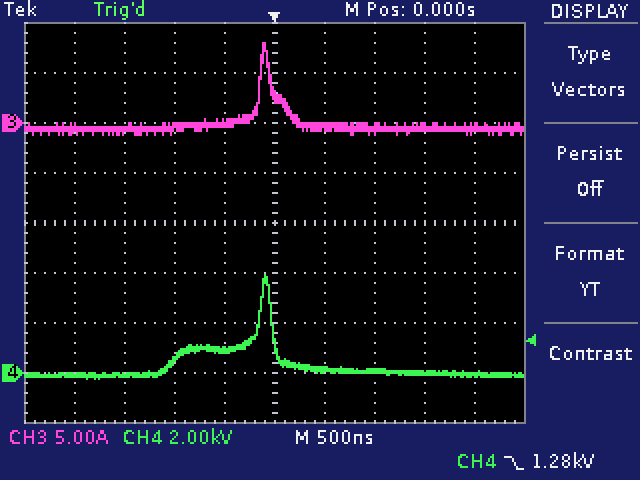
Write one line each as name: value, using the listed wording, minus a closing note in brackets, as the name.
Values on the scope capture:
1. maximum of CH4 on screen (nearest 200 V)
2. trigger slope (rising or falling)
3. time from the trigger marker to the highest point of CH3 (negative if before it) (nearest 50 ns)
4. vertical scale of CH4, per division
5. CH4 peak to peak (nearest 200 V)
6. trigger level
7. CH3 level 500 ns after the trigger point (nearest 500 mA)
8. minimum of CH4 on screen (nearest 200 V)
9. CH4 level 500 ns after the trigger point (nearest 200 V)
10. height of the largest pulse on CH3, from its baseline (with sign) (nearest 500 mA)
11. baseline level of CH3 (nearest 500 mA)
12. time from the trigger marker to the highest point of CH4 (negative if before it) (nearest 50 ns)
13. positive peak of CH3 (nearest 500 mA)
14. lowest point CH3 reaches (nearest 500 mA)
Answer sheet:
maximum of CH4 on screen: 4.0 kV
trigger slope: falling
time from the trigger marker to the highest point of CH3 (negative if before it): -100 ns
vertical scale of CH4, per division: 2 kV
CH4 peak to peak: 4.2 kV
trigger level: 1.28 kV
CH3 level 500 ns after the trigger point: -500 mA
minimum of CH4 on screen: -200 V
CH4 level 500 ns after the trigger point: 200 V
height of the largest pulse on CH3, from its baseline (with sign): +8.5 A
baseline level of CH3: -500 mA
time from the trigger marker to the highest point of CH4 (negative if before it): -100 ns
positive peak of CH3: 8.0 A
lowest point CH3 reaches: -1.0 A
